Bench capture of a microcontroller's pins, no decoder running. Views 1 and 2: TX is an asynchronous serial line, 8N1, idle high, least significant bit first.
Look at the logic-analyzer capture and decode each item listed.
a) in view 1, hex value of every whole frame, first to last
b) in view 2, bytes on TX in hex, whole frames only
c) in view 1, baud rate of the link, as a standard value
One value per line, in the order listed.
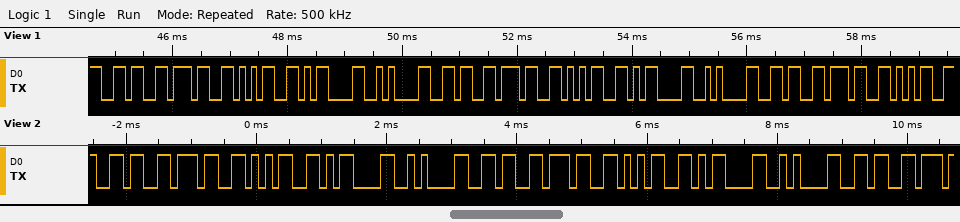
0x36 0x37 0x35 0x0D 0x0A 0x36 0x37 0x35 0x0D 0x0A 0x36 0x37 0x35
36 37 35 0D 0A 36 37 35 0D 0A 36
9600 baud
